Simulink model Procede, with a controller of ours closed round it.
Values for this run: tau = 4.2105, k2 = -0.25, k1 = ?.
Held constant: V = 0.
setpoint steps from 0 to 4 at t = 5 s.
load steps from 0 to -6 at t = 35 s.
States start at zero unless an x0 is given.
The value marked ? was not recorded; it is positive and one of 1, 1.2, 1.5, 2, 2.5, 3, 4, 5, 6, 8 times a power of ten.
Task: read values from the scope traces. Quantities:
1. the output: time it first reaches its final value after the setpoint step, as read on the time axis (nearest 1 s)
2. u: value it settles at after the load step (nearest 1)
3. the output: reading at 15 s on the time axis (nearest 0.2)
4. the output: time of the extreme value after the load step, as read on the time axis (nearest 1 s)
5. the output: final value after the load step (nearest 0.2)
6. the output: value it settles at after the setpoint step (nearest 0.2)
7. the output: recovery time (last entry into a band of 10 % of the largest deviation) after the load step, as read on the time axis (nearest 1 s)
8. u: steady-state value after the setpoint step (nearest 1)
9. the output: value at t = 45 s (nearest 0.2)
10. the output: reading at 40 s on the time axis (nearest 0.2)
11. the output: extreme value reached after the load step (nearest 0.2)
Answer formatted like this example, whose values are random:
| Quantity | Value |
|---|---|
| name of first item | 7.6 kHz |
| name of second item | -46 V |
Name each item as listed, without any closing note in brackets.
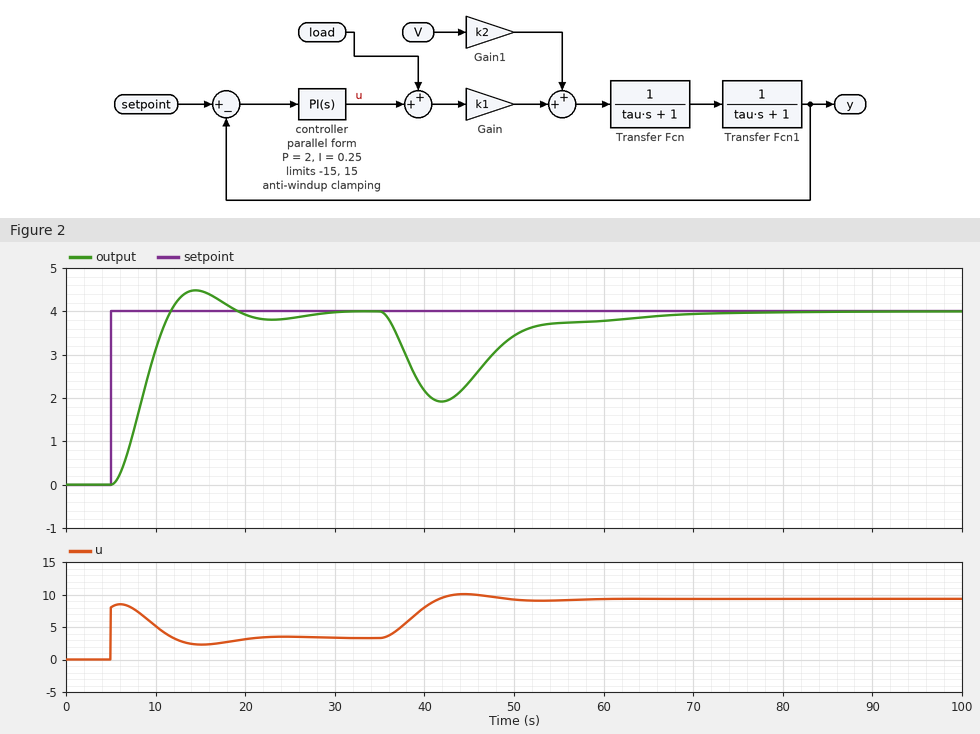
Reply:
| Quantity | Value |
|---|---|
| the output: time it first reaches its final value after the setpoint step, as read on the time axis | 12 s |
| u: value it settles at after the load step | 9 |
| the output: reading at 15 s on the time axis | 4.4 |
| the output: time of the extreme value after the load step, as read on the time axis | 42 s |
| the output: final value after the load step | 4.0 |
| the output: value it settles at after the setpoint step | 4.0 |
| the output: recovery time (last entry into a band of 10 % of the largest deviation) after the load step, as read on the time axis | 61 s |
| u: steady-state value after the setpoint step | 3 |
| the output: value at t = 45 s | 2.4 |
| the output: reading at 40 s on the time axis | 2.2 |
| the output: extreme value reached after the load step | 2.0 |
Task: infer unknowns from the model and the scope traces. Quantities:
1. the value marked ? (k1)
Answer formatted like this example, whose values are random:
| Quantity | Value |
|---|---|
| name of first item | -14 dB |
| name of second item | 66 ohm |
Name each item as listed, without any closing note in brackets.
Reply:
| Quantity | Value |
|---|---|
| the value marked ? | 1.2 |
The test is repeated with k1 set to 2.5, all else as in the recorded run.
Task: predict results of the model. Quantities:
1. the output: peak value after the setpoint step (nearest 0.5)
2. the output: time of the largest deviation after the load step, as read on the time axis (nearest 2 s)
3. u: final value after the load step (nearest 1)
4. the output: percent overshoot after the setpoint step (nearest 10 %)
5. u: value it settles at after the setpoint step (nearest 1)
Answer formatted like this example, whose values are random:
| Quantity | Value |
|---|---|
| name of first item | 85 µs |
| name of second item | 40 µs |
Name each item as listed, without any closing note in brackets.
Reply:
| Quantity | Value |
|---|---|
| the output: peak value after the setpoint step | 5.0 |
| the output: time of the largest deviation after the load step, as read on the time axis | 40 s |
| u: final value after the load step | 8 |
| the output: percent overshoot after the setpoint step | 30 % |
| u: value it settles at after the setpoint step | 2 |
